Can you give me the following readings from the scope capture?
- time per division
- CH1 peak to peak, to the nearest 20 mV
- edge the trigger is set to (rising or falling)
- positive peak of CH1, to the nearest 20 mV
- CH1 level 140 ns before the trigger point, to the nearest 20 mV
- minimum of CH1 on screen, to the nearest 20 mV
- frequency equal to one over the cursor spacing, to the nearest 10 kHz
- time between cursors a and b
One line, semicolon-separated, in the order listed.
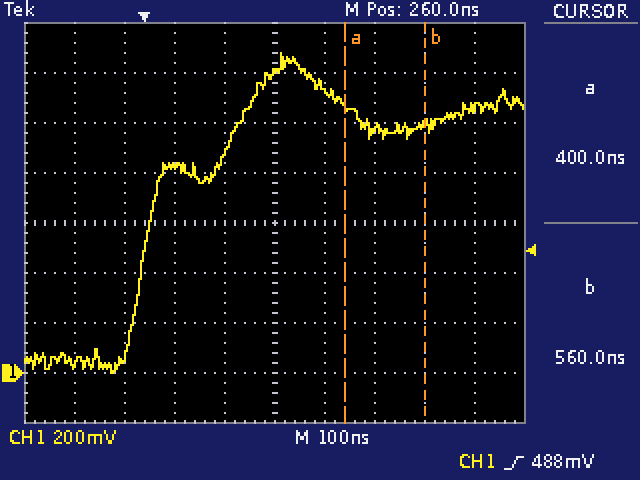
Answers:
100 ns; 1.28 V; rising; 1.28 V; 40 mV; 0 mV; 6.25 MHz; 160 ns
